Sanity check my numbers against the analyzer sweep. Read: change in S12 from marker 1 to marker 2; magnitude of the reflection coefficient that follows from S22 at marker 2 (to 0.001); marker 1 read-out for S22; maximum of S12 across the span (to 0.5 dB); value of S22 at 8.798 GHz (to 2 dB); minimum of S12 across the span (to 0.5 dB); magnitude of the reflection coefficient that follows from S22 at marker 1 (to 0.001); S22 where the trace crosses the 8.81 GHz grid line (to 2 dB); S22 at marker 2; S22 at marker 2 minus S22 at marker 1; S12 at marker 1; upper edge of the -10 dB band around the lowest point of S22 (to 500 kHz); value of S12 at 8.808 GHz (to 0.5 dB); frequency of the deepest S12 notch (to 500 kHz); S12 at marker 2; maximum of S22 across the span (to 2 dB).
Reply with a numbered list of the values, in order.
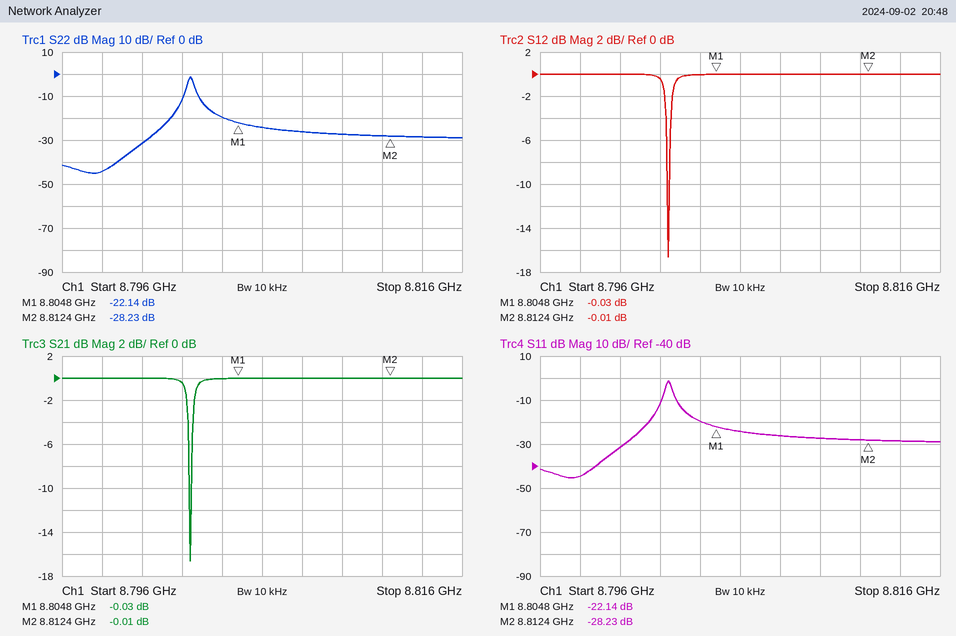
1. 0.02 dB
2. 0.039
3. -22.14 dB
4. 0.0 dB
5. -44 dB
6. -16.5 dB
7. 0.078
8. -28 dB
9. -28.23 dB
10. -6.09 dB
11. -0.03 dB
12. 8.8020 GHz
13. 0.0 dB
14. 8.8025 GHz
15. -0.01 dB
16. -2 dB
